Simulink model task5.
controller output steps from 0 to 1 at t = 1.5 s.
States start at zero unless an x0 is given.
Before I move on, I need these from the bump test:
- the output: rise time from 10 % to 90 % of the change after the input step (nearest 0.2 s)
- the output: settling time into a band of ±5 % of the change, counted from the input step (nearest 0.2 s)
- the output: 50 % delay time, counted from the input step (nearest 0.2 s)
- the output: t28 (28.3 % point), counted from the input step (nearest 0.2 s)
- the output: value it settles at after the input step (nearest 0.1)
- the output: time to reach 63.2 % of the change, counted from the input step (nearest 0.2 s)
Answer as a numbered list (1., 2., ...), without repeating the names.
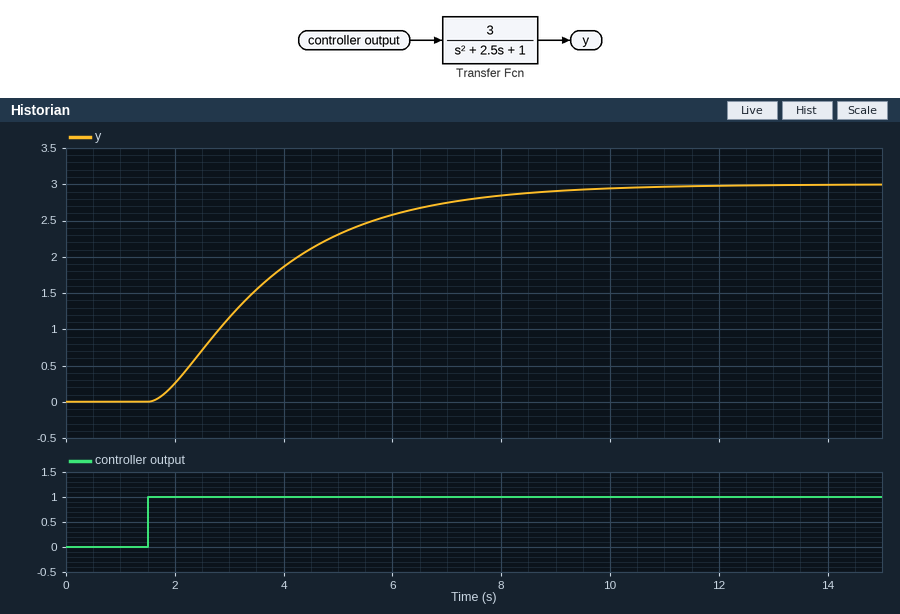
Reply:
1. 4.6 s
2. 6.6 s
3. 2.0 s
4. 1.2 s
5. 3.0
6. 2.6 s
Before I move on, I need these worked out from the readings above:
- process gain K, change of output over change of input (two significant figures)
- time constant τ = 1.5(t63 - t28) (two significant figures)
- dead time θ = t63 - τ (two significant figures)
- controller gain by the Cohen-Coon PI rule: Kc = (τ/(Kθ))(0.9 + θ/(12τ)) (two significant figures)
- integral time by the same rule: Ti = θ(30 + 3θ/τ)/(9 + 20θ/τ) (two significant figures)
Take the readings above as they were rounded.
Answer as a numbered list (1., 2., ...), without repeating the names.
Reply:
1. 3.0
2. 2.1 s
3. 0.50 s
4. 1.3
5. 1.1 s
